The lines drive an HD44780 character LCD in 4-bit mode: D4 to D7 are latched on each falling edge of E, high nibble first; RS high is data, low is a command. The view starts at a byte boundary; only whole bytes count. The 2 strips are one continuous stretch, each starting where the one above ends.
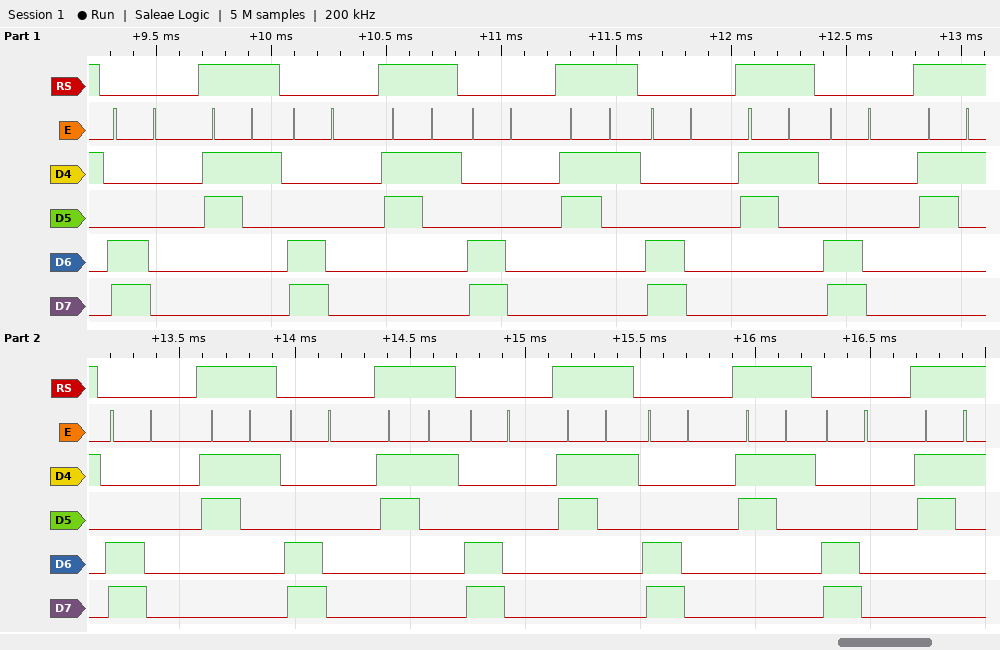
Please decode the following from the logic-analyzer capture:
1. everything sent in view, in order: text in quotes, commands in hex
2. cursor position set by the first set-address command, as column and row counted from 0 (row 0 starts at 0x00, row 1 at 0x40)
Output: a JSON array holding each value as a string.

["0xC0 \"1\" 0xC0 \"1\" 0xC0 \"1\" 0xC0 \"1\" 0xC0 \"1\" 0xC0 \"1\" 0xC0 \"1\" 0xC0 \"1\" 0xC0 \"1\" 0xC0 \"1\"", "column 0, row 1"]
